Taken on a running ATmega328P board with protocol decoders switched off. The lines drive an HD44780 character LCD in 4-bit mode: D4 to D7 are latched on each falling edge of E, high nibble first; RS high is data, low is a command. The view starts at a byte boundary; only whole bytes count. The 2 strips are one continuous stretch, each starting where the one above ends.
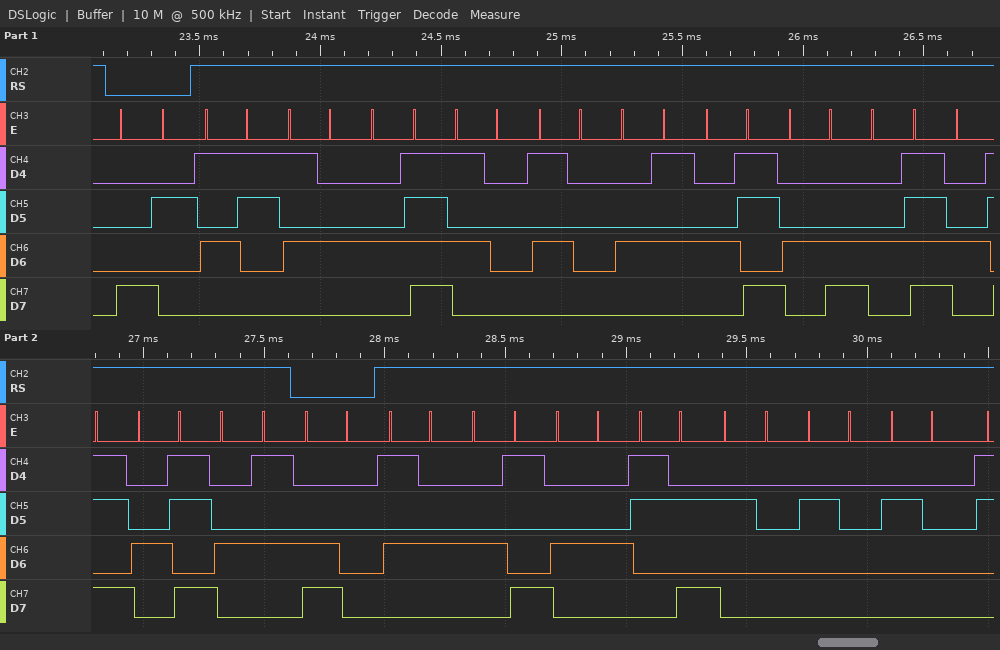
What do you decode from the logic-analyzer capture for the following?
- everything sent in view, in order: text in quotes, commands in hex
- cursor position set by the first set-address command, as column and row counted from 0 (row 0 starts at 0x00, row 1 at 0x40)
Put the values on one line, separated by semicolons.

0x82 "STOPPEKLOKKE" 0xC0 "TID:   "; column 2, row 0
